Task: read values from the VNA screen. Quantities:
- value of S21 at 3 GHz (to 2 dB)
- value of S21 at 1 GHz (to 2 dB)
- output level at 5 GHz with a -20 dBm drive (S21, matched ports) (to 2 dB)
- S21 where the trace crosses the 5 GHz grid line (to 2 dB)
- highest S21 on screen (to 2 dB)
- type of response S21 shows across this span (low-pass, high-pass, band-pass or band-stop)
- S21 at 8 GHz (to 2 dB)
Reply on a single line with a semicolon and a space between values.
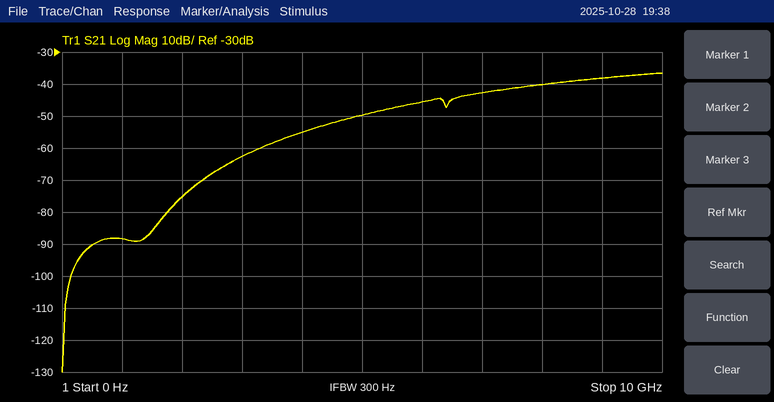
-62 dB; -88 dB; -70 dBm; -50 dB; -36 dB; high-pass; -40 dB
